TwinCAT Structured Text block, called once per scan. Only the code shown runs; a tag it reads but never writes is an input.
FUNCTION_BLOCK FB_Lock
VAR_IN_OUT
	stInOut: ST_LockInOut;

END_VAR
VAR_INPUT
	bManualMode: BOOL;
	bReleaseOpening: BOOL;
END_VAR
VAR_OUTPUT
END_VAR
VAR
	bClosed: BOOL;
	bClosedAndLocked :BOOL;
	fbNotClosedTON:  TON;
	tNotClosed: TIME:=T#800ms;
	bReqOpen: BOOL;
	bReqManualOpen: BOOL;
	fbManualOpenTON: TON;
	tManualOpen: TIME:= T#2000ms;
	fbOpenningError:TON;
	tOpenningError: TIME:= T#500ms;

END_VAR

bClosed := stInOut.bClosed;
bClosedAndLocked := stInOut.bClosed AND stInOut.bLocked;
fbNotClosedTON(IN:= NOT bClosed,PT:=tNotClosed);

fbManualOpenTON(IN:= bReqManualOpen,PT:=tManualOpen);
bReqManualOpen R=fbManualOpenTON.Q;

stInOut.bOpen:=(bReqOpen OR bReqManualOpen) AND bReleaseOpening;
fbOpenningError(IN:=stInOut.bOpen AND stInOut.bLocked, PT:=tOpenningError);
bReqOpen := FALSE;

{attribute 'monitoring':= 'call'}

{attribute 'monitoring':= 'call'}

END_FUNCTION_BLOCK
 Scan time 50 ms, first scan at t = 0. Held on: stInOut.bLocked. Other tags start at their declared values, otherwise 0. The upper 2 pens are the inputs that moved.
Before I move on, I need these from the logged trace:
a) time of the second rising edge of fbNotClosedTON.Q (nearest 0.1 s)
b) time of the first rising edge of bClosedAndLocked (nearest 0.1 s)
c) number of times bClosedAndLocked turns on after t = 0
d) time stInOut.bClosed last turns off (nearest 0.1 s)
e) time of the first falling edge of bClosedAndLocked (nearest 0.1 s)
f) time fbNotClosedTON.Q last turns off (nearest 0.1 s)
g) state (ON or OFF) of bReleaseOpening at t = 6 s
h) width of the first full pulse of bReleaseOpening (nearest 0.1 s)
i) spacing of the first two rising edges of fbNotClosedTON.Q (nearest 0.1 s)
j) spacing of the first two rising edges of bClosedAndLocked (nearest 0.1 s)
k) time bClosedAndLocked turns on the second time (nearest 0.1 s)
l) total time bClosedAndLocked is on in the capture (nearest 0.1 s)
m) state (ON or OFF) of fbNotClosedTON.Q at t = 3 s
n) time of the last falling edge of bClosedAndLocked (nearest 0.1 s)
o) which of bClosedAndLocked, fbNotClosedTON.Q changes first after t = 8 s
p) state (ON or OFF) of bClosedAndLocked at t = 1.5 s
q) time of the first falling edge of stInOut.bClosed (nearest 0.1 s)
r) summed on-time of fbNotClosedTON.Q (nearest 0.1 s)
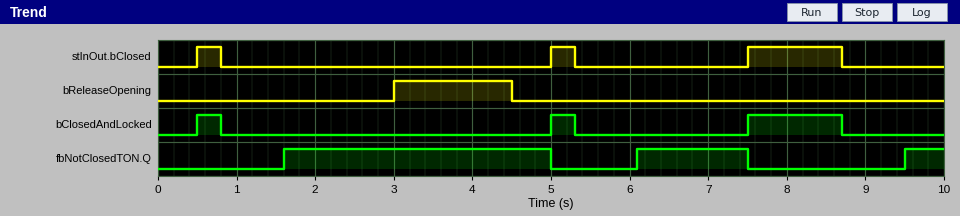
6.1 s
0.5 s
3
8.7 s
0.8 s
7.5 s
OFF
1.5 s
4.5 s
4.5 s
5.0 s
1.8 s
ON
8.7 s
bClosedAndLocked
OFF
0.8 s
5.3 s
